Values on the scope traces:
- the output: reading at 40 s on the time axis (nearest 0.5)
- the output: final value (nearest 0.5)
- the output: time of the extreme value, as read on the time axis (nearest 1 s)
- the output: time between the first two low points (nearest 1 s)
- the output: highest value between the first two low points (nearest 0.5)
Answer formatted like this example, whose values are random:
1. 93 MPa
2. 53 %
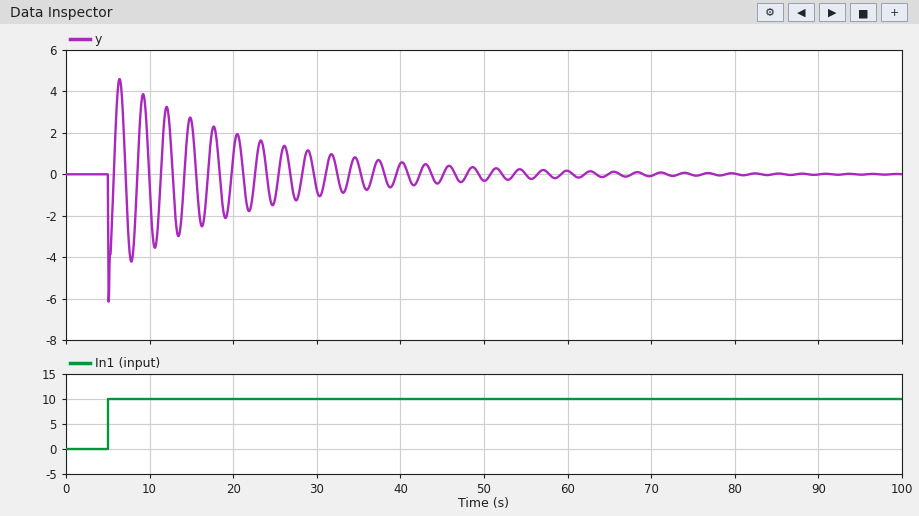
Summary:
1. 0.5
2. 0.0
3. 5 s
4. 3 s
5. 4.5
